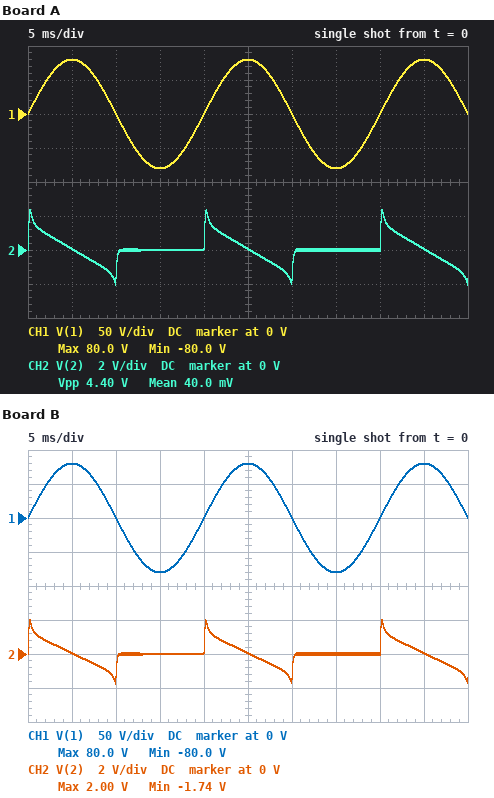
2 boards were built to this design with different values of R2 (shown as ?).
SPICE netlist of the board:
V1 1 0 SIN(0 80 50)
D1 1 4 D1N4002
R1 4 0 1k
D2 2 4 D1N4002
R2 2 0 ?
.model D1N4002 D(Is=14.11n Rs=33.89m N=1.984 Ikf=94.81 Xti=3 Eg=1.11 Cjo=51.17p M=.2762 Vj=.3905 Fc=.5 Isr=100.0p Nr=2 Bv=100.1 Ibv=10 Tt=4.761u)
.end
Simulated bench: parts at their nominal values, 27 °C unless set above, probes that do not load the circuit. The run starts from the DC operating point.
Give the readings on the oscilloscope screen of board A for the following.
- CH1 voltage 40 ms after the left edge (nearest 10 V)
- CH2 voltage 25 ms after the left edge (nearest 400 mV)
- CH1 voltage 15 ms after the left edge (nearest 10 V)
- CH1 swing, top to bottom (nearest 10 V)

0 V
0 V
-80 V
160 V
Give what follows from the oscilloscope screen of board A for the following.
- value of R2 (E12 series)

3.3 MΩ
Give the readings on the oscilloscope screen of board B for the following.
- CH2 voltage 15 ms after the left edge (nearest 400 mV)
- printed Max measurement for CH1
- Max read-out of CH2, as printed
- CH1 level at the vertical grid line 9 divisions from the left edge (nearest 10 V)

0 V
80.0 V
2.00 V
80 V
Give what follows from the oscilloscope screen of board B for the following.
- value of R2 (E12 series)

2.7 MΩ
